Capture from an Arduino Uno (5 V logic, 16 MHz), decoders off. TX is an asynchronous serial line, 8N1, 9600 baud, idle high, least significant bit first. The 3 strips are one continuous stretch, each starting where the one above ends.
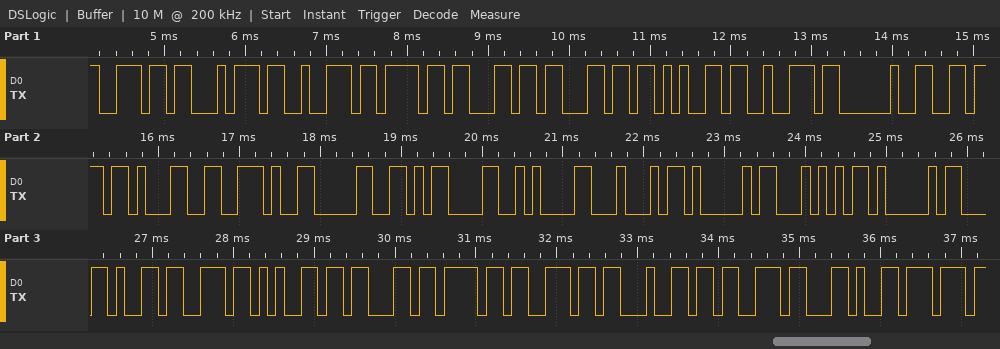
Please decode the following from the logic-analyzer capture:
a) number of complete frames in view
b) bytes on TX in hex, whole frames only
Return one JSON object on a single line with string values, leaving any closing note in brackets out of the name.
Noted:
{"number of complete frames in view": "29", "bytes on TX in hex, whole frames only": "0x6E 0x74 0x72 0x6F 0x6C 0x6C 0x65 0x72 0x20 0x76 0x31 0x2E 0x30 0x0D 0x0A 0x44 0x41 0x54 0x41 0x2C 0x73 0x65 0x63 0x6F 0x6E 0x64 0x73 0x2C 0x77"}
